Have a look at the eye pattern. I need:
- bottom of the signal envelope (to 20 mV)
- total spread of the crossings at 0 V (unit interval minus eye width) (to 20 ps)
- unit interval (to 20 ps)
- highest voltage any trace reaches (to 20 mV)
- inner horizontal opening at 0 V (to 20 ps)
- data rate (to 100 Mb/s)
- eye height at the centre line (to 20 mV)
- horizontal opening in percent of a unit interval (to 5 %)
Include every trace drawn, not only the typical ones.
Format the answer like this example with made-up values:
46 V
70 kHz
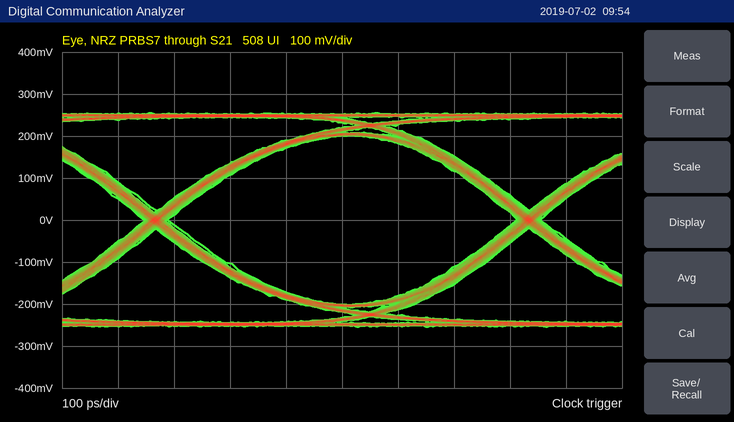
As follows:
-260 mV
40 ps
660 ps
260 mV
620 ps
1.5 Gb/s
400 mV
95 %
